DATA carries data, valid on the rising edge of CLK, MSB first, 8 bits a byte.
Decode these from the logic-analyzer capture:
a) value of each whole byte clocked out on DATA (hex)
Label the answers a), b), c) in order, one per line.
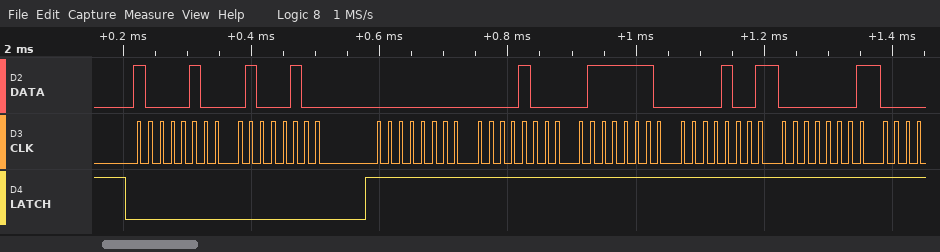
a) 84 44 00 08 7E 09 01
